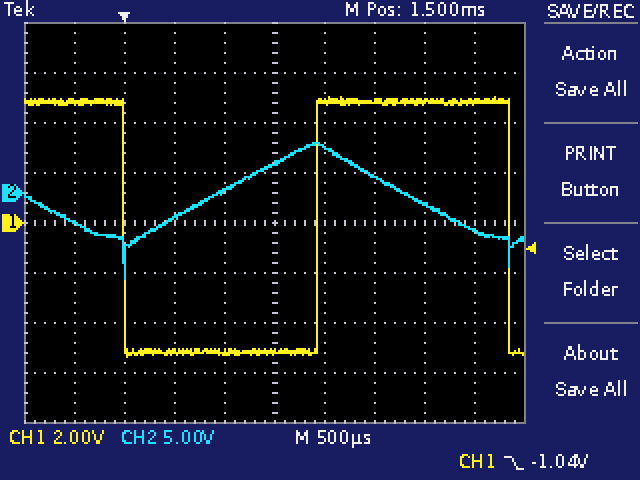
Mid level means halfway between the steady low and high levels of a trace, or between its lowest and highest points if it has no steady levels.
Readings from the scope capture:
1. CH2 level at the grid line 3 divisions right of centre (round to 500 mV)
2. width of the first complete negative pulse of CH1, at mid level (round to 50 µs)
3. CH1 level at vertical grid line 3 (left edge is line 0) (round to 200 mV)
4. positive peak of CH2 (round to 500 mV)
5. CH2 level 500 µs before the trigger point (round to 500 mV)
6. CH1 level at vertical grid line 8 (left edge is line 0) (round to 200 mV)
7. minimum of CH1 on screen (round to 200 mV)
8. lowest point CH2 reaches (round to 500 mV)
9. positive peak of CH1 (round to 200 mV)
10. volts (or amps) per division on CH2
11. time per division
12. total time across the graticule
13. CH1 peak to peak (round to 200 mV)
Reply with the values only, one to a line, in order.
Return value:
-1.0 V
1.95 ms
-5.2 V
5.0 V
-3.0 V
4.8 V
-5.4 V
-8.5 V
5.0 V
5 V
500 µs
5 ms
10.4 V
